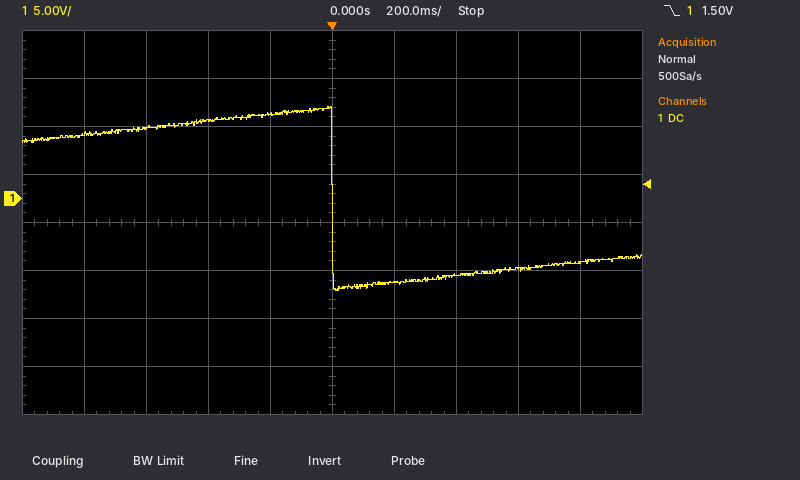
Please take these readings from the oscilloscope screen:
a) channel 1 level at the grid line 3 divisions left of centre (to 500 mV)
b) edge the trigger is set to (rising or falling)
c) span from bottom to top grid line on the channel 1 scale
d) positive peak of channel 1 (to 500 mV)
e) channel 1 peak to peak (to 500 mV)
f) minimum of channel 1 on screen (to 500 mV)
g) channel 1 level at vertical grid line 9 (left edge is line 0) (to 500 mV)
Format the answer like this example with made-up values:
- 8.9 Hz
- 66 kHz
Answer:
- 7.5 V
- falling
- 40 V
- 9.5 V
- 19.0 V
- -9.5 V
- -6.5 V
